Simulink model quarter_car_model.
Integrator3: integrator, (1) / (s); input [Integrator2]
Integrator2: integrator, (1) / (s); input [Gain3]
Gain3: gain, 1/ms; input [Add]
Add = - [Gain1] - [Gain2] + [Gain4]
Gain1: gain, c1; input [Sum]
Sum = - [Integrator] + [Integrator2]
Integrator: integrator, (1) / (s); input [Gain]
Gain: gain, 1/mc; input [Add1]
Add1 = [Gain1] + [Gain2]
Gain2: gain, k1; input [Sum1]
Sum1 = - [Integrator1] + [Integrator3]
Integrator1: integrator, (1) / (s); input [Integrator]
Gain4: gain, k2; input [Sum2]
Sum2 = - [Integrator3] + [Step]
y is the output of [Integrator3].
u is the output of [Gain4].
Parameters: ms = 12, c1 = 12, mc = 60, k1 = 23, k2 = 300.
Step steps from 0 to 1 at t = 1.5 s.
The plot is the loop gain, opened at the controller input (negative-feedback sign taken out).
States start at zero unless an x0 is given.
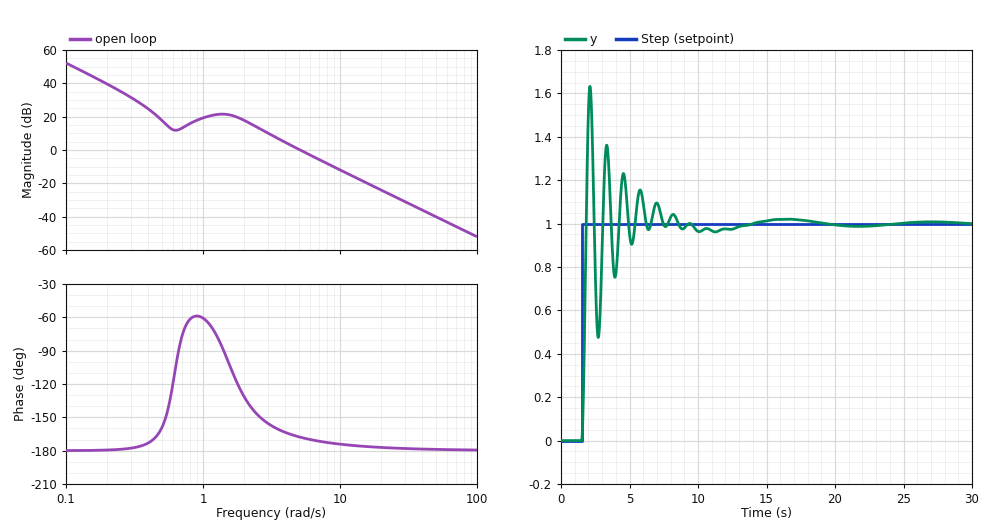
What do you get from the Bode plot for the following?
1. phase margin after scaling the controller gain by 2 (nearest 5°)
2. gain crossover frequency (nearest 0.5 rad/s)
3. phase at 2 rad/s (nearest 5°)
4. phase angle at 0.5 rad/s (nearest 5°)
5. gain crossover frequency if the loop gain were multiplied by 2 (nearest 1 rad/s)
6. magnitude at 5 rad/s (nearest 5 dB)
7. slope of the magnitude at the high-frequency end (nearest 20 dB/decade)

10°
5.0 rad/s
-130°
-160°
7 rad/s
0 dB
-40 dB/decade
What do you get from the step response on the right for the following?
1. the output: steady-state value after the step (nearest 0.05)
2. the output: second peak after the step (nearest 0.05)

1.00
1.35
